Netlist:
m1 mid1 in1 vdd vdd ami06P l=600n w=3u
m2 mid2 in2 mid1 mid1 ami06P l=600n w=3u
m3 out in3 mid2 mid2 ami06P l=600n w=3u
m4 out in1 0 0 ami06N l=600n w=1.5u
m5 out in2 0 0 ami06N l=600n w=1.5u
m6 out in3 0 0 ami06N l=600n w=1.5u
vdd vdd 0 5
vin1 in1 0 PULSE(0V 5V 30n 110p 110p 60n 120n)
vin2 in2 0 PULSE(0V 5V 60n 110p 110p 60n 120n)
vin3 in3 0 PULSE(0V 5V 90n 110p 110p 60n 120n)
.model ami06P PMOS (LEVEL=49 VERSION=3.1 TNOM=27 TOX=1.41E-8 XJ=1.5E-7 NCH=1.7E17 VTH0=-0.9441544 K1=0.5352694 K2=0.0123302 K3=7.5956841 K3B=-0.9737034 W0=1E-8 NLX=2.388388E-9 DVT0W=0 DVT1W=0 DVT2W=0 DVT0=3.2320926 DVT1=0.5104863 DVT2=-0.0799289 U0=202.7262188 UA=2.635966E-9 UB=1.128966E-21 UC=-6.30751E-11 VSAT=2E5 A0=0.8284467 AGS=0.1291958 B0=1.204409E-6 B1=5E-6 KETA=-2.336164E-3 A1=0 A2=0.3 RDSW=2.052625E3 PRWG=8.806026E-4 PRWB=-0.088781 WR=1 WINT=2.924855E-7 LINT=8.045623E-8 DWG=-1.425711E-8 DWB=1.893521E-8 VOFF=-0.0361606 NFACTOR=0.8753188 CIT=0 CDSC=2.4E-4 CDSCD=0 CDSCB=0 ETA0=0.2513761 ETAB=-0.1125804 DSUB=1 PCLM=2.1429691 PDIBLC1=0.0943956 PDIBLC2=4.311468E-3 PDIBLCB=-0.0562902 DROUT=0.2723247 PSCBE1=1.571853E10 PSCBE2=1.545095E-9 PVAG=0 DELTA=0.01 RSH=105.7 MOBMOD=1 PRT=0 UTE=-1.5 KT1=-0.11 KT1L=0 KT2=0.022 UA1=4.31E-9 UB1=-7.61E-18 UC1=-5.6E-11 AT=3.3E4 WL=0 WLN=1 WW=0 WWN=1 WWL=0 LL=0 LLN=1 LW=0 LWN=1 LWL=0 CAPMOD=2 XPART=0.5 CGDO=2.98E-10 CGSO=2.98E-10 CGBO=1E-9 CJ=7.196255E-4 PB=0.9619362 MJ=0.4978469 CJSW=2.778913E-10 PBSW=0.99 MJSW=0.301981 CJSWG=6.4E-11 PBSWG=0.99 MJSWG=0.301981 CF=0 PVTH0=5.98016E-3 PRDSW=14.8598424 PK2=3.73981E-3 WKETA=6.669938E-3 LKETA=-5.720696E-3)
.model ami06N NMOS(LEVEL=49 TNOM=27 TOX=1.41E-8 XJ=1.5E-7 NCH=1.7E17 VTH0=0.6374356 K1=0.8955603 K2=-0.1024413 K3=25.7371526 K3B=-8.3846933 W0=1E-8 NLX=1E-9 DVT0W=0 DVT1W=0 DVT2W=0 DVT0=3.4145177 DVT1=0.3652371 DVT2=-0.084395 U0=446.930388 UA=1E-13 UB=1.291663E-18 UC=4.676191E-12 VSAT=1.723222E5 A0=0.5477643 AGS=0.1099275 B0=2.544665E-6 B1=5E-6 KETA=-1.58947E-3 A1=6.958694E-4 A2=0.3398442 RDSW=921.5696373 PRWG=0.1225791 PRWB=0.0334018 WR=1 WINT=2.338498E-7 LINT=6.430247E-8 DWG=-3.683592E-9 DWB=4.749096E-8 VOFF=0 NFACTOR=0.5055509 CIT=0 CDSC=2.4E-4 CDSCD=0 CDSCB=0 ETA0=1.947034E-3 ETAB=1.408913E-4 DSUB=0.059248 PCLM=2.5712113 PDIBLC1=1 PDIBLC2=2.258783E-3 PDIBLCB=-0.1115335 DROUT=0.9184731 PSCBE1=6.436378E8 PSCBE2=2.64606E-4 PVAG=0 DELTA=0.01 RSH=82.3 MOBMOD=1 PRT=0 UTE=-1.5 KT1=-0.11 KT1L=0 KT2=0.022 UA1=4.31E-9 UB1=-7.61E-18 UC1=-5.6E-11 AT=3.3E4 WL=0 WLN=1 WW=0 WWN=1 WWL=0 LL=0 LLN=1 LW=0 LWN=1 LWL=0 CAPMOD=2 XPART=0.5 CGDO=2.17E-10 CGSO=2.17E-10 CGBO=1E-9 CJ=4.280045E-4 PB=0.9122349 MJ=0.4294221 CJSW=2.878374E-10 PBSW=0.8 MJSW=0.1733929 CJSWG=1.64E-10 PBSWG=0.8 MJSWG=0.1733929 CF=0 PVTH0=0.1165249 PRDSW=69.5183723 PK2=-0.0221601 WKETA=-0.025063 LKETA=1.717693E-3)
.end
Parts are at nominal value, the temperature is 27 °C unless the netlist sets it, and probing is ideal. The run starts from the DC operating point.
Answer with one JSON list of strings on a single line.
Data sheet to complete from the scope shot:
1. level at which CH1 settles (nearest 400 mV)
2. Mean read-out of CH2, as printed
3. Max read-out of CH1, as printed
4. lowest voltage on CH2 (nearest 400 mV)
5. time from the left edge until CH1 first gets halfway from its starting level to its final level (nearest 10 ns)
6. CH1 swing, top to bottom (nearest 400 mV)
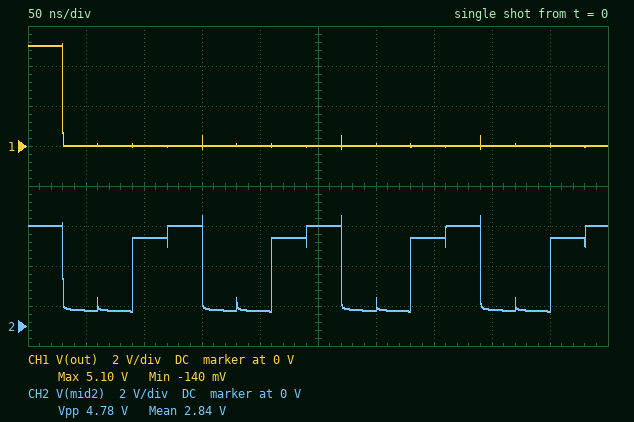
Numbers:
["0 V", "2.84 V", "5.10 V", "800 mV", "30 ns", "5.2 V"]
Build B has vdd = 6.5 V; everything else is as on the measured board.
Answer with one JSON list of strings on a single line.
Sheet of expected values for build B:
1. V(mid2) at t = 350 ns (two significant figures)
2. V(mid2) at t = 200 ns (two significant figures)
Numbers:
["6.2 V", "1.3 V"]
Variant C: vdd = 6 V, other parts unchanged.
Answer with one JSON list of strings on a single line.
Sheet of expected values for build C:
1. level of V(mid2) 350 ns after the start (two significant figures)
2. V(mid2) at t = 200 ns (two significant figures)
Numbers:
["5.9 V", "970 mV"]
